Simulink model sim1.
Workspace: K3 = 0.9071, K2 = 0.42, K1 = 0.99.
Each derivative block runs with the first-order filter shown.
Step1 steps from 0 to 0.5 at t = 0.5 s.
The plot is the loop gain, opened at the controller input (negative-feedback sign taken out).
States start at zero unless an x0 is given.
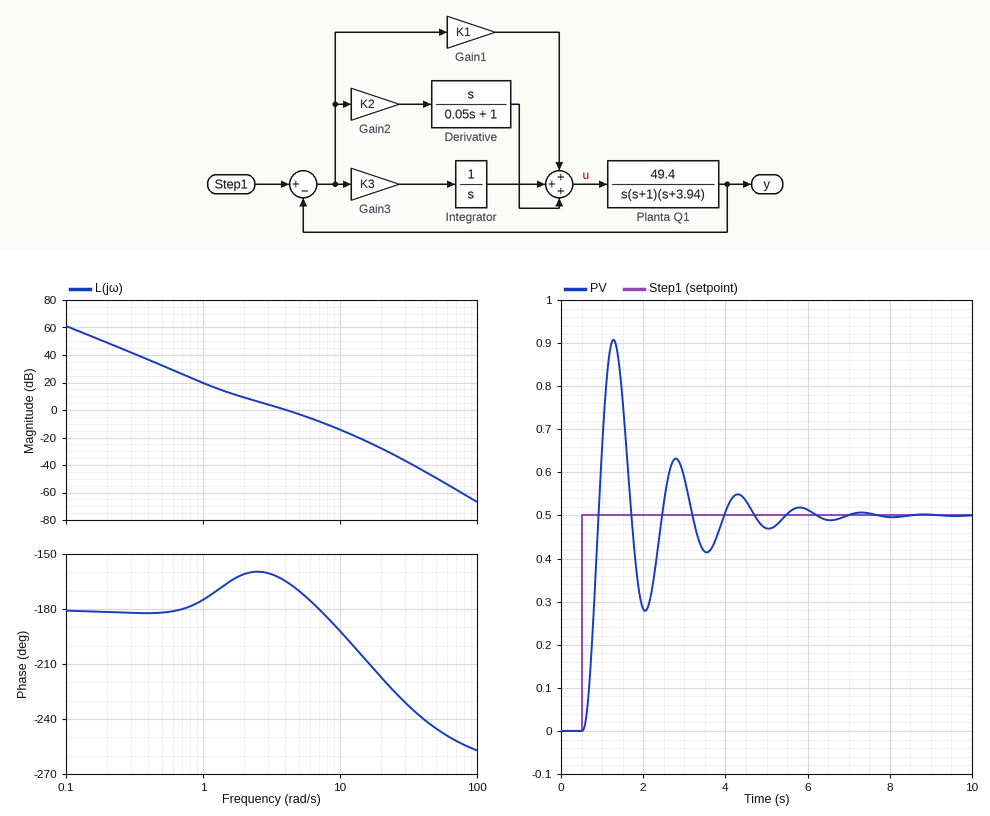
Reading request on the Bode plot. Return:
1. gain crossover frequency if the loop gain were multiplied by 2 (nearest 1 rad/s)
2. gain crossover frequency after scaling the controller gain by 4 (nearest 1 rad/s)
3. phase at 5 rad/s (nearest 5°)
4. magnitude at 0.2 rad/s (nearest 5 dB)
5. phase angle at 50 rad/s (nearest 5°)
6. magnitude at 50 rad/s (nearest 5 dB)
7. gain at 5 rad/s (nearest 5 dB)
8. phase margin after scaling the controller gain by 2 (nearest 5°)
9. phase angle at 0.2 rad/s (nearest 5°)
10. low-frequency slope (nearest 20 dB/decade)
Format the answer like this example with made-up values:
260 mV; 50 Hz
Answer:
6 rad/s; 9 rad/s; -170°; 50 dB; -245°; -50 dB; -5 dB; 5°; -180°; -40 dB/decade
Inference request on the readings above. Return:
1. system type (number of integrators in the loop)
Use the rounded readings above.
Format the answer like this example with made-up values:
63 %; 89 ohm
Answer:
2
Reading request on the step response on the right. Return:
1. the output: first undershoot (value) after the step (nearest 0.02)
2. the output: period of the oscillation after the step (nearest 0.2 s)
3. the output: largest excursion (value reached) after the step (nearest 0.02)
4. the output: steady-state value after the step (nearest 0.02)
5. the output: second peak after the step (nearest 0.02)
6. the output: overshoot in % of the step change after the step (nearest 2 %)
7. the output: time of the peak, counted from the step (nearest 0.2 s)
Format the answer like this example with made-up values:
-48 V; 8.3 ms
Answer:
0.28; 1.6 s; 0.90; 0.50; 0.64; 82 %; 0.8 s
